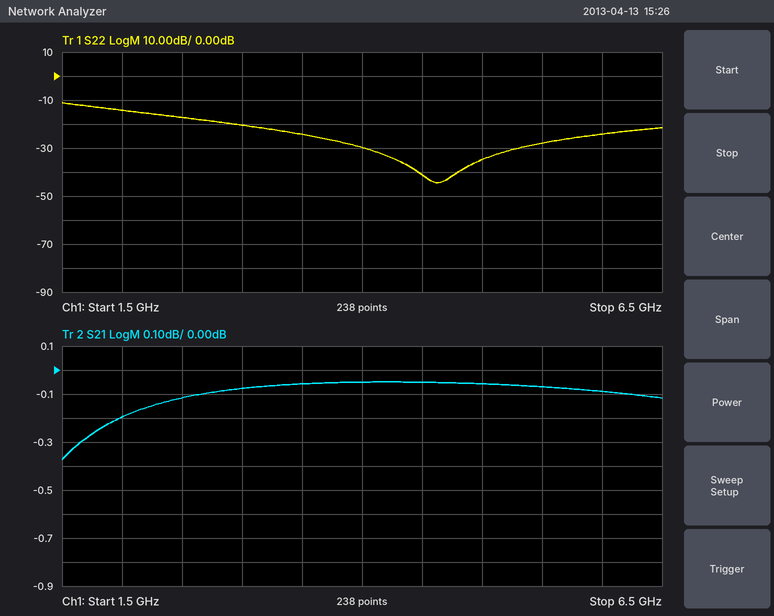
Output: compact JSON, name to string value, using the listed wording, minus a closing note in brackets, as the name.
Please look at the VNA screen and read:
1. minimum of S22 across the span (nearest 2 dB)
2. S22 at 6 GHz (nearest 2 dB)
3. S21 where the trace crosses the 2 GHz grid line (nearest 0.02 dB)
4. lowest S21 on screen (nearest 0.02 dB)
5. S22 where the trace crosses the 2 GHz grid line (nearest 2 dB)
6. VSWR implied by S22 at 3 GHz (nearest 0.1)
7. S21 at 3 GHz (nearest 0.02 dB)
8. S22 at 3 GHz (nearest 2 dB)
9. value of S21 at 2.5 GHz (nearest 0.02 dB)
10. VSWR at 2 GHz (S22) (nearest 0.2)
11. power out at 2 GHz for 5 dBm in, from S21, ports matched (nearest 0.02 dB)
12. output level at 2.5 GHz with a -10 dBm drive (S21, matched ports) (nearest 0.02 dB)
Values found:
{"minimum of S22 across the span": "-44 dB", "S22 at 6 GHz": "-24 dB", "S21 where the trace crosses the 2 GHz grid line": "-0.20 dB", "lowest S21 on screen": "-0.38 dB", "S22 where the trace crosses the 2 GHz grid line": "-14 dB", "VSWR implied by S22 at 3 GHz": "1.2", "S21 at 3 GHz": "-0.08 dB", "S22 at 3 GHz": "-20 dB", "value of S21 at 2.5 GHz": "-0.12 dB", "VSWR at 2 GHz (S22)": "1.4", "power out at 2 GHz for 5 dBm in, from S21, ports matched": "4.80 dBm", "output level at 2.5 GHz with a -10 dBm drive (S21, matched ports)": "-10.12 dBm"}
